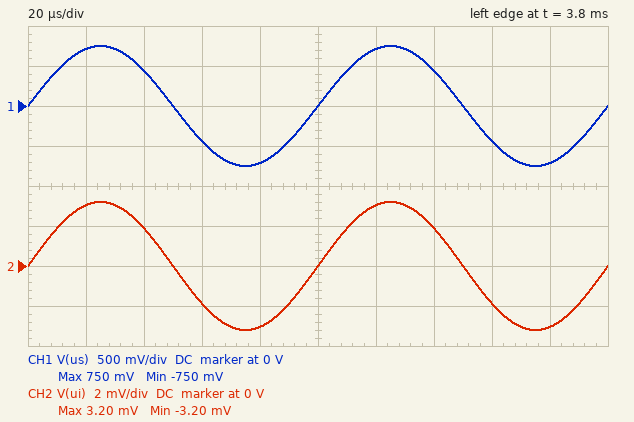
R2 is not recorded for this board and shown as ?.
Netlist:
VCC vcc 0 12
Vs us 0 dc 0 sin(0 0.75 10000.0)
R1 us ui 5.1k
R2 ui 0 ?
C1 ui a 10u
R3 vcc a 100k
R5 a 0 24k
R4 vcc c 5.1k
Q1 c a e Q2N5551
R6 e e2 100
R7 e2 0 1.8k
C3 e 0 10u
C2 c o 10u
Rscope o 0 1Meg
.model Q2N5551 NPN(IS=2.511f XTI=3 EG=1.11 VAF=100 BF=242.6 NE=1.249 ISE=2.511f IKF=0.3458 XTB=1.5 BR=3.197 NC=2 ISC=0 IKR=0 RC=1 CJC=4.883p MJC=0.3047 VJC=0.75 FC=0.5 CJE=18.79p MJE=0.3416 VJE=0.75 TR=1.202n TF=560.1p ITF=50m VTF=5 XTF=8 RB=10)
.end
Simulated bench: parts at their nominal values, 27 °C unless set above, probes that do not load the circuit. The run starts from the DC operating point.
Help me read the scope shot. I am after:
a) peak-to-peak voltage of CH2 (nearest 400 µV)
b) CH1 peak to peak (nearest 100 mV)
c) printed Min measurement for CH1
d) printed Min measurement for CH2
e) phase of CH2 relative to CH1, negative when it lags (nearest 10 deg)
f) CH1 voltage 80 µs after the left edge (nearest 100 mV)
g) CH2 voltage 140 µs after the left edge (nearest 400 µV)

6.4 mV
1.5 V
-750 mV
-3.20 mV
0 deg
-700 mV
2.0 mV
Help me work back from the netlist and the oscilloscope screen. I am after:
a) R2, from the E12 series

22 Ω
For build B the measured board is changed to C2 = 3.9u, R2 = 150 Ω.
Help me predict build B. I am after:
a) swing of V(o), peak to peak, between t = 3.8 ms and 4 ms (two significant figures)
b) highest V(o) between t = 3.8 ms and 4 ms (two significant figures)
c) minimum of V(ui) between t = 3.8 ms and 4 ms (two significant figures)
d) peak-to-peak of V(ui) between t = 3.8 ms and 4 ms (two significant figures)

5.8 V
2.4 V
-21 mV
41 mV
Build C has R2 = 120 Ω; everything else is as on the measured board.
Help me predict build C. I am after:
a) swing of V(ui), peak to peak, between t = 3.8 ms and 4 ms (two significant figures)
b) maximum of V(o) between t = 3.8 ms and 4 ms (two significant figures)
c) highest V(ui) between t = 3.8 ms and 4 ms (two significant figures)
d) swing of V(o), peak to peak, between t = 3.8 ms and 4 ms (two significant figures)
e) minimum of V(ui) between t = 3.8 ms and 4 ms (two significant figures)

33 mV
2.0 V
17 mV
4.8 V
-17 mV
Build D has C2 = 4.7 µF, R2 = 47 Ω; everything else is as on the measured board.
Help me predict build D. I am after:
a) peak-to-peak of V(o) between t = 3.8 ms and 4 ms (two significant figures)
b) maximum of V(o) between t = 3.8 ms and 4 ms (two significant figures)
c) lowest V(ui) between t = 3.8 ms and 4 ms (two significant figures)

2.0 V
930 mV
-6.8 mV
